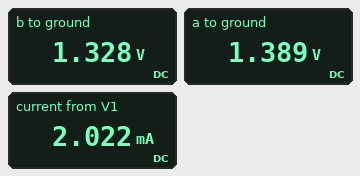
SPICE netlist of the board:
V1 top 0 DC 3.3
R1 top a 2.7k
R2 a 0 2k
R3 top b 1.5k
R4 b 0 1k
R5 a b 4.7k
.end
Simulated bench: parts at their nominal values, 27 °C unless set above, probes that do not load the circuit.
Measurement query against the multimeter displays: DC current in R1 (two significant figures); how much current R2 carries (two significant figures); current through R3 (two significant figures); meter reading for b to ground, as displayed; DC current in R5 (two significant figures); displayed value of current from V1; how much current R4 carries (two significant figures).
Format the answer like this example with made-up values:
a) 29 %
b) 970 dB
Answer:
a) 710 µA
b) 690 µA
c) 1.3 mA
d) 1.328 V
e) 13 µA
f) 2.022 mA
g) 1.3 mA
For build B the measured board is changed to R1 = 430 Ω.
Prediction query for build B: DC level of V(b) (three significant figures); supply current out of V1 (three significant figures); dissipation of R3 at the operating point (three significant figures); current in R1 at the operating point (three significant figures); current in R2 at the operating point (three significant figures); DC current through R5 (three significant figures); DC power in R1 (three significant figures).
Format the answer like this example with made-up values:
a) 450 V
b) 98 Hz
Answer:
a) 1.47 V
b) 2.78 mA
c) 2.24 mW
d) 1.56 mA
e) 1.31 mA
f) 247 µA
g) 1.05 mW
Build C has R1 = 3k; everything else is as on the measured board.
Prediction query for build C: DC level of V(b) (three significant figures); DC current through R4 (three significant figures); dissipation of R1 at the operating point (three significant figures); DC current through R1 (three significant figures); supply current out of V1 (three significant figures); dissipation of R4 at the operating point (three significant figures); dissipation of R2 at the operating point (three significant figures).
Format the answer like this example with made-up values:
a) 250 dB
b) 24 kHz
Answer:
a) 1.32 V
b) 1.32 mA
c) 1.31 mW
d) 660 µA
e) 1.98 mA
f) 1.74 mW
g) 871 µW
